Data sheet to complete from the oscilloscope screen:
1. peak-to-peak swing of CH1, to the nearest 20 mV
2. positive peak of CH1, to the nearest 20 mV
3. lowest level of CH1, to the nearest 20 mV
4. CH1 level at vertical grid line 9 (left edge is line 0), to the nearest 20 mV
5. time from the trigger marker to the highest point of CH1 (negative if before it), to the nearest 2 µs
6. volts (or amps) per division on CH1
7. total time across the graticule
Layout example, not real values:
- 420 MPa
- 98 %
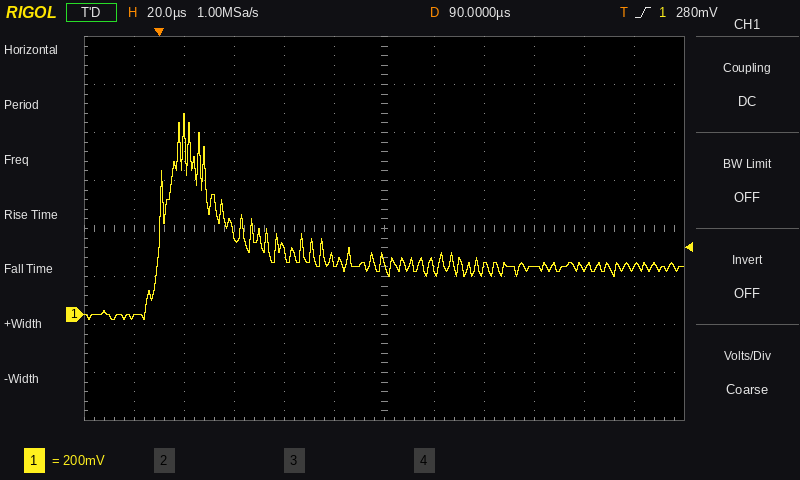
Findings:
- 860 mV
- 840 mV
- -20 mV
- 200 mV
- +10 µs
- 200 mV
- 240 µs
